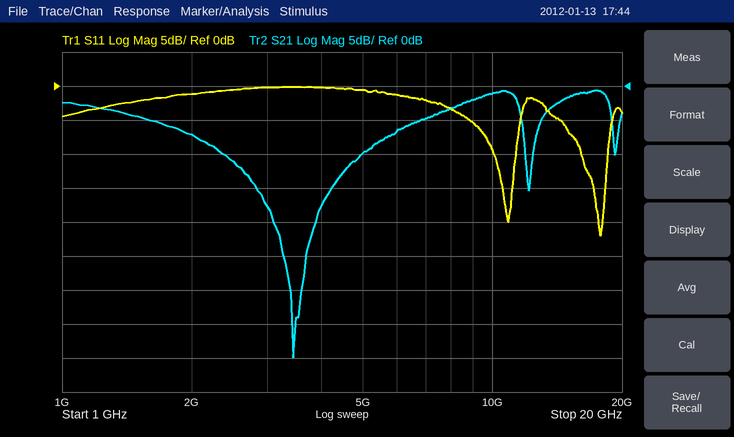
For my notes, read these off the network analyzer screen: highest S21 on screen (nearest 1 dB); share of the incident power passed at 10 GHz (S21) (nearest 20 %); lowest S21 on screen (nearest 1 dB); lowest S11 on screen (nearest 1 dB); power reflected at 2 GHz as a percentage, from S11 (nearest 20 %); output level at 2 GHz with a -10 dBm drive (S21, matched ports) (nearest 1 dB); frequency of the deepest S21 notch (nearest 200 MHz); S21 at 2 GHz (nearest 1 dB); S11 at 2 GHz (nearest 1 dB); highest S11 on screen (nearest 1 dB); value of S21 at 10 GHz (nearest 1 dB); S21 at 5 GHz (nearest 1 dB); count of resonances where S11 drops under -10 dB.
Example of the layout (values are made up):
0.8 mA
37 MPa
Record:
-1 dB
80 %
-40 dB
-22 dB
80 %
-17 dBm
3.4 GHz
-7 dB
-1 dB
0 dB
-1 dB
-10 dB
2
